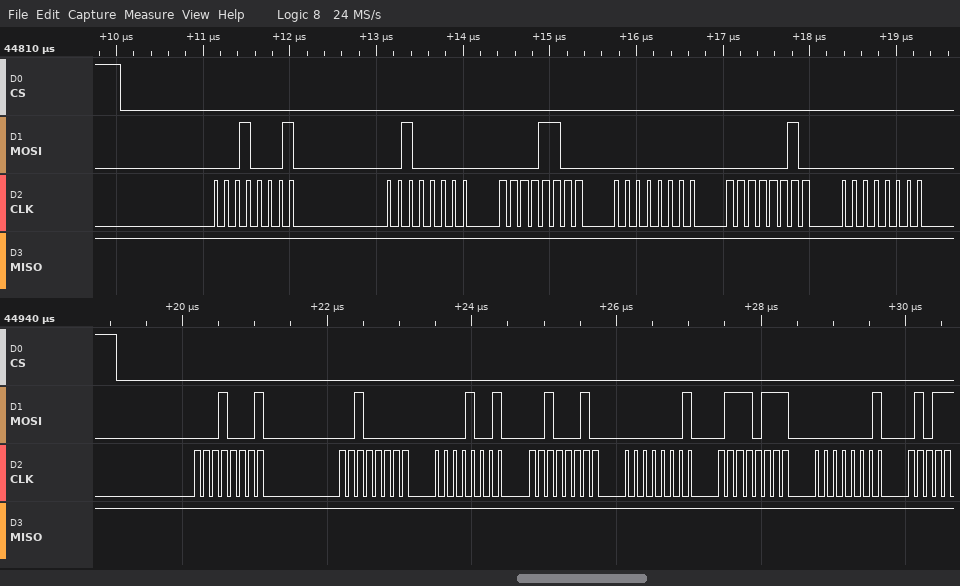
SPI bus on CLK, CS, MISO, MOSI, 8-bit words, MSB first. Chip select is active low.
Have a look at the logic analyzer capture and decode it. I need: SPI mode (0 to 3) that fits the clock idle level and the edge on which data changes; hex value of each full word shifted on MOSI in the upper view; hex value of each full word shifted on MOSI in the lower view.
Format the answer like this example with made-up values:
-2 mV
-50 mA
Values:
0
11, 20, 0C, 00, 02, 00
11, 20, 09, 22, 01, 77, 01
